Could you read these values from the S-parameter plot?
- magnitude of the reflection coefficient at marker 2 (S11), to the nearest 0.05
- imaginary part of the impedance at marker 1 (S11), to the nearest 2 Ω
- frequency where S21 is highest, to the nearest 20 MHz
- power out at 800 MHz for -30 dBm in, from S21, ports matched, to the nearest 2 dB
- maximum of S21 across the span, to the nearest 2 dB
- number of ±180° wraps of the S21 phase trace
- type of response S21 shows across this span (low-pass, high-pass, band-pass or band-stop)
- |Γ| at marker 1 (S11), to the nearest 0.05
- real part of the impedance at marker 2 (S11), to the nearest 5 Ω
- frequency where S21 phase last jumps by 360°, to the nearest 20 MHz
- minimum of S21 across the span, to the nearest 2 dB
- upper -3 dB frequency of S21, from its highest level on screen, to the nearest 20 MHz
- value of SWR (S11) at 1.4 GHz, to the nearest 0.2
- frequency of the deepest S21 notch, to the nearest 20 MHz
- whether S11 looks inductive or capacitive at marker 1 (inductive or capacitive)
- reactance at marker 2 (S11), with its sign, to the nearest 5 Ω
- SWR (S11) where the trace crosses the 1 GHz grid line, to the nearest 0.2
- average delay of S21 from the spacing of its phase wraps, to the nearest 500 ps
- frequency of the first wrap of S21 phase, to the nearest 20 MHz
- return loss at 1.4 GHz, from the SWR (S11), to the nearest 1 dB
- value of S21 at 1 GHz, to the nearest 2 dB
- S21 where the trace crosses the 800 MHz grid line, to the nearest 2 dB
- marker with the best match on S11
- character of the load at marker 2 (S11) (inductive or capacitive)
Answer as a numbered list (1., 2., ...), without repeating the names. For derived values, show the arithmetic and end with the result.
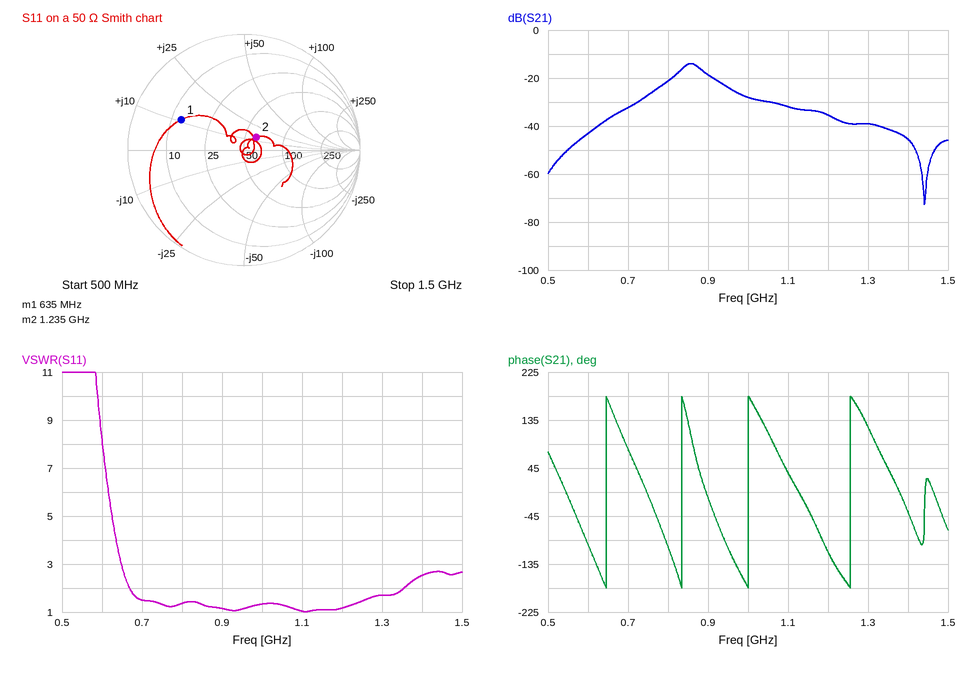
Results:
1. 0.15
2. +10 Ω
3. 860 MHz
4. -30 dBm + (-22 dB) = -52 dBm
5. -14 dB
6. 4
7. band-pass
8. 0.60
9. 60 Ω
10. 1.26 GHz
11. -72 dB
12. 880 MHz
13. 2.6
14. 1.44 GHz
15. inductive
16. +15 Ω
17. 1.4
18. 3 cycles / (1.26 GHz − 640 MHz) ≈ 4.84 ns, so 5.0 ns to the nearest 500 ps
19. 640 MHz
20. −20 log10((2.6 − 1)/(2.6 + 1)) ≈ 7 dB
21. -28 dB
22. -22 dB
23. marker 2
24. inductive
